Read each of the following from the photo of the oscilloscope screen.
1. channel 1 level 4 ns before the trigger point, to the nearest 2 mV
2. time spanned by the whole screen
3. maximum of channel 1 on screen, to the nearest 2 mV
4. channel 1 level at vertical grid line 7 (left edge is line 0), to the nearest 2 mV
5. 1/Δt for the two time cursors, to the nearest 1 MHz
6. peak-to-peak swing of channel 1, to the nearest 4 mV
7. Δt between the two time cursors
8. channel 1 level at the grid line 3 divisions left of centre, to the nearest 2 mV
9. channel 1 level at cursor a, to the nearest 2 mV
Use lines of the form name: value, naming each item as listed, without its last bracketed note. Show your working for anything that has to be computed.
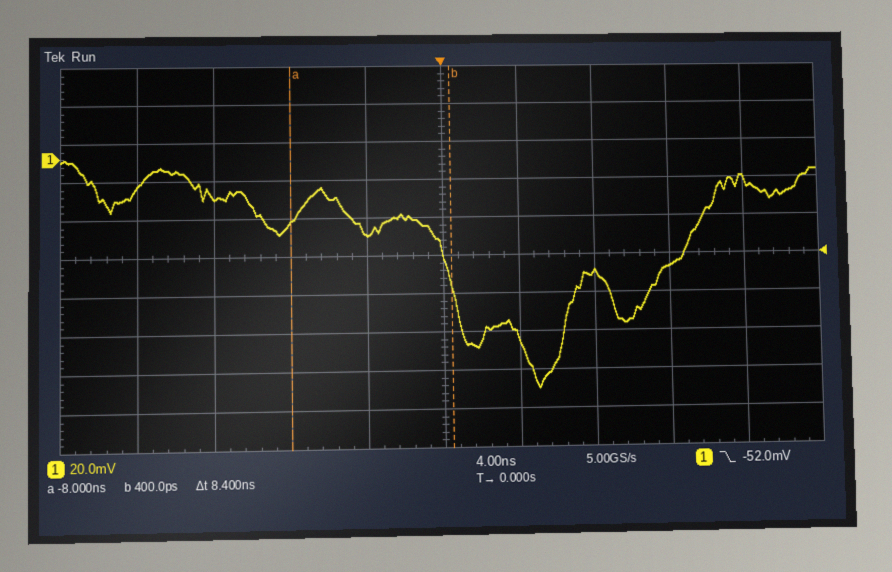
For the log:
channel 1 level 4 ns before the trigger point, to the nearest 2 mV: -40 mV
time spanned by the whole screen: 40 ns
maximum of channel 1 on screen, to the nearest 2 mV: 0 mV
channel 1 level at vertical grid line 7 (left edge is line 0), to the nearest 2 mV: -62 mV
1/Δt for the two time cursors, to the nearest 1 MHz: 1 / 8.4 ns ≈ 119 MHz
peak-to-peak swing of channel 1, to the nearest 4 mV: 120 mV
Δt between the two time cursors: 8.4 ns
channel 1 level at the grid line 3 divisions left of centre, to the nearest 2 mV: -20 mV
channel 1 level at cursor a, to the nearest 2 mV: -34 mV
